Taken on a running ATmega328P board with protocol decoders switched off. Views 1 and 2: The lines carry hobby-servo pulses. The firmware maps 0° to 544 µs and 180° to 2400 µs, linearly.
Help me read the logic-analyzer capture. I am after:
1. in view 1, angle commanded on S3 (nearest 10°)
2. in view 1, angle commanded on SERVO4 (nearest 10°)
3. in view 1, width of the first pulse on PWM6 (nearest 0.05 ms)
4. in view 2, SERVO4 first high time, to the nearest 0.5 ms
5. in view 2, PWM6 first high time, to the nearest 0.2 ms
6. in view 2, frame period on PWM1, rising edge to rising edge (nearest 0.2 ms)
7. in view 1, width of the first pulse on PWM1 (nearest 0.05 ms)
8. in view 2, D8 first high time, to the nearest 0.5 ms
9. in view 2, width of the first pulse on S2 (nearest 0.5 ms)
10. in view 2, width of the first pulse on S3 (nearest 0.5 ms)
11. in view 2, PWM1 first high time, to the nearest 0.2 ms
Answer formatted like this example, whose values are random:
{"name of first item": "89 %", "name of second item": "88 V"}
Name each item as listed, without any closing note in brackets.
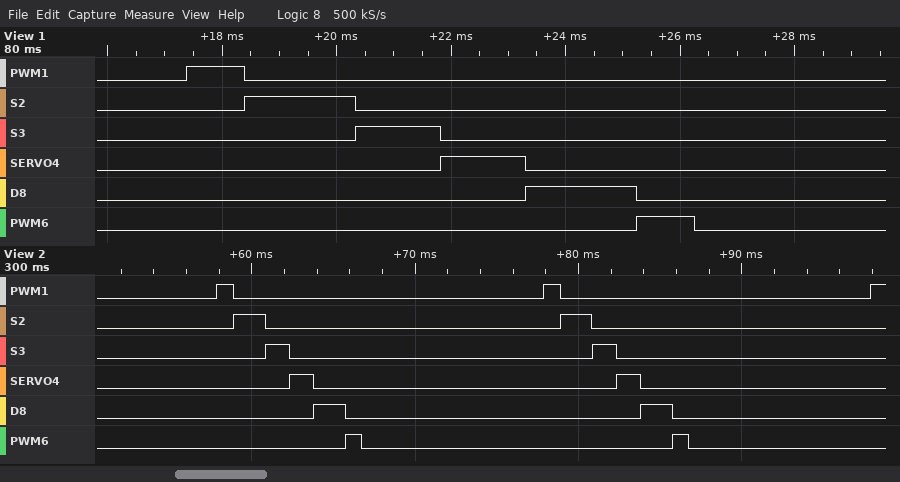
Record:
{"in view 1, angle commanded on S3": "90°", "in view 1, angle commanded on SERVO4": "90°", "in view 1, width of the first pulse on PWM6": "1.00 ms", "in view 2, SERVO4 first high time, to the nearest 0.5 ms": "1.5 ms", "in view 2, PWM6 first high time, to the nearest 0.2 ms": "1.0 ms", "in view 2, frame period on PWM1, rising edge to rising edge": "20.0 ms", "in view 1, width of the first pulse on PWM1": "1.00 ms", "in view 2, D8 first high time, to the nearest 0.5 ms": "2.0 ms", "in view 2, width of the first pulse on S2": "2.0 ms", "in view 2, width of the first pulse on S3": "1.5 ms", "in view 2, PWM1 first high time, to the nearest 0.2 ms": "1.0 ms"}
